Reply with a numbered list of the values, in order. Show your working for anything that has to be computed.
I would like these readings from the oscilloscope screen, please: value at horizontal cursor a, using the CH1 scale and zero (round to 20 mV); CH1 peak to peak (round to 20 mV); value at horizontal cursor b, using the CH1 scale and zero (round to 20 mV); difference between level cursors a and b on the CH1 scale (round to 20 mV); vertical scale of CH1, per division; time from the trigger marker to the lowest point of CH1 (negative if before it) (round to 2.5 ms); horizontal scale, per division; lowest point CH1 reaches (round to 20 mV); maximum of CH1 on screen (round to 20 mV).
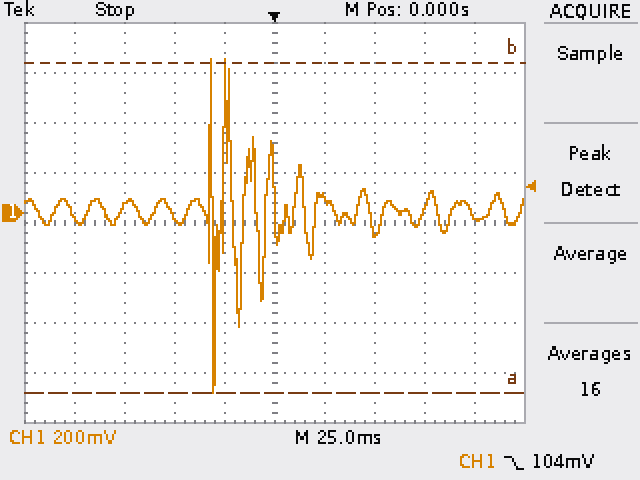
1. -720 mV
2. 620 mV − (-720 mV) = 1.34 V
3. 600 mV
4. 1.32 V
5. 200 mV
6. -30.0 ms
7. 25 ms
8. -720 mV
9. 620 mV
